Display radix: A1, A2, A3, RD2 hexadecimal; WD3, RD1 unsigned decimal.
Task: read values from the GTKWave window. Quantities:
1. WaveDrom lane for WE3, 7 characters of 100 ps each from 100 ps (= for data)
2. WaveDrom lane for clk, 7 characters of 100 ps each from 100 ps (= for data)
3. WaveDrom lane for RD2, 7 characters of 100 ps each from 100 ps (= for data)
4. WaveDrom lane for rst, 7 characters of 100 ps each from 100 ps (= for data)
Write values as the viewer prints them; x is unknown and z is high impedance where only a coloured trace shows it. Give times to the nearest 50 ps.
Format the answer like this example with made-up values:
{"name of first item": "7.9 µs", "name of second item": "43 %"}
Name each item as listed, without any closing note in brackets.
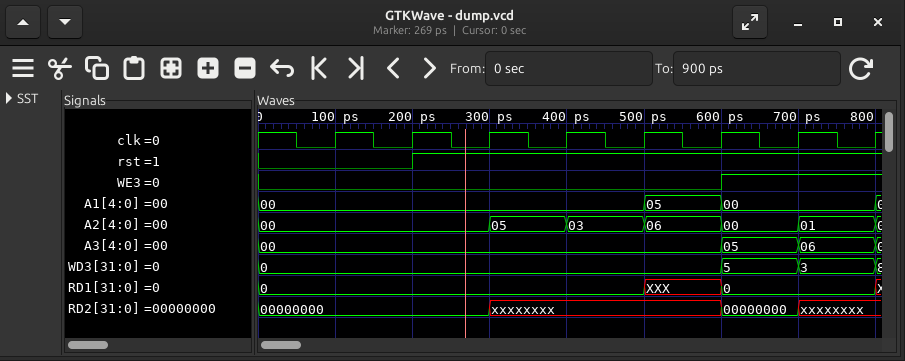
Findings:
{"WaveDrom lane for WE3, 7 characters of 100 ps each from 100 ps": "{name: 'WE3', wave: '0....1.'}", "WaveDrom lane for clk, 7 characters of 100 ps each from 100 ps": "{name: 'clk', wave: 'p......'}", "WaveDrom lane for RD2, 7 characters of 100 ps each from 100 ps": "{name: 'RD2', wave: '=.x..=x', data: '00000000 00000000'}", "WaveDrom lane for rst, 7 characters of 100 ps each from 100 ps": "{name: 'rst', wave: '01.....'}"}
